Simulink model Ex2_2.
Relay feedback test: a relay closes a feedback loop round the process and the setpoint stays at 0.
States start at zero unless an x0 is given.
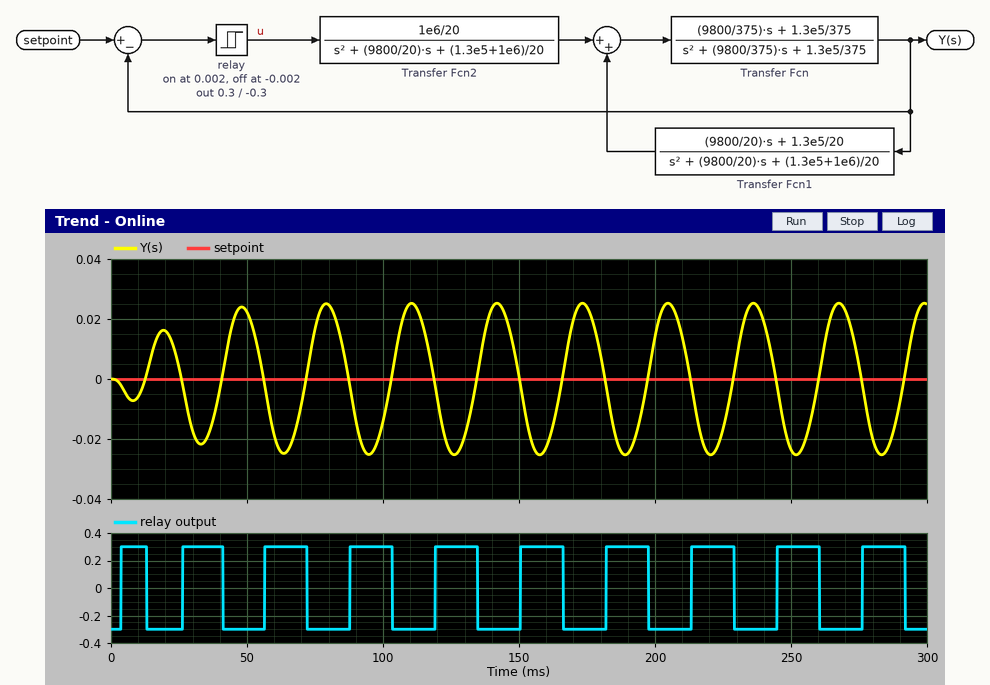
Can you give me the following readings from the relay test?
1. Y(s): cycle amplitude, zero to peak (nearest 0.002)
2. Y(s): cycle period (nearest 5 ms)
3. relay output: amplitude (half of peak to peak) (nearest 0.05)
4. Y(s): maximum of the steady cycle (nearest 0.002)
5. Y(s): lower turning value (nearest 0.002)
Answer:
0.026
30 ms
0.30
0.026
-0.026
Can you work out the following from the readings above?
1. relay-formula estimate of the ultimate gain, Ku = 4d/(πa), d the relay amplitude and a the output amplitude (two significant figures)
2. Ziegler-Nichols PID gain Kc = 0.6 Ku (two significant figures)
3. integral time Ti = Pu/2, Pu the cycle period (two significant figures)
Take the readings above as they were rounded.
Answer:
15
9.0
15 ms
